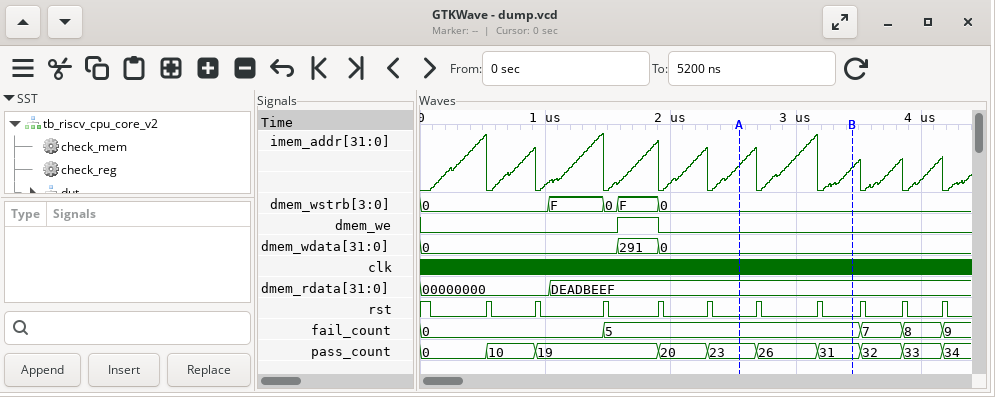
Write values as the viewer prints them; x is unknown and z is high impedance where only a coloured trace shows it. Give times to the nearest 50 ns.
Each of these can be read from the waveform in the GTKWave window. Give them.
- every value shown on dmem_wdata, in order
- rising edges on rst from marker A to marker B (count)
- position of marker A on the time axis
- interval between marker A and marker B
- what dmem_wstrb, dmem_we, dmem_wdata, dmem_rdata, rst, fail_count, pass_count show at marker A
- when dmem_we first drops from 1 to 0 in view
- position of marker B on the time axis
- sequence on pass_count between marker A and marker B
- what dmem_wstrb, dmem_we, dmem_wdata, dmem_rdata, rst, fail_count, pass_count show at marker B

0, 291, 0
2
2550 ns
900 ns
dmem_wstrb=0, dmem_we=0, dmem_wdata=0, dmem_rdata=DEADBEEF, rst=0, fail_count=5, pass_count=23
1900 ns
3450 ns
23, 26, 31
dmem_wstrb=0, dmem_we=0, dmem_wdata=0, dmem_rdata=DEADBEEF, rst=0, fail_count=5, pass_count=31
